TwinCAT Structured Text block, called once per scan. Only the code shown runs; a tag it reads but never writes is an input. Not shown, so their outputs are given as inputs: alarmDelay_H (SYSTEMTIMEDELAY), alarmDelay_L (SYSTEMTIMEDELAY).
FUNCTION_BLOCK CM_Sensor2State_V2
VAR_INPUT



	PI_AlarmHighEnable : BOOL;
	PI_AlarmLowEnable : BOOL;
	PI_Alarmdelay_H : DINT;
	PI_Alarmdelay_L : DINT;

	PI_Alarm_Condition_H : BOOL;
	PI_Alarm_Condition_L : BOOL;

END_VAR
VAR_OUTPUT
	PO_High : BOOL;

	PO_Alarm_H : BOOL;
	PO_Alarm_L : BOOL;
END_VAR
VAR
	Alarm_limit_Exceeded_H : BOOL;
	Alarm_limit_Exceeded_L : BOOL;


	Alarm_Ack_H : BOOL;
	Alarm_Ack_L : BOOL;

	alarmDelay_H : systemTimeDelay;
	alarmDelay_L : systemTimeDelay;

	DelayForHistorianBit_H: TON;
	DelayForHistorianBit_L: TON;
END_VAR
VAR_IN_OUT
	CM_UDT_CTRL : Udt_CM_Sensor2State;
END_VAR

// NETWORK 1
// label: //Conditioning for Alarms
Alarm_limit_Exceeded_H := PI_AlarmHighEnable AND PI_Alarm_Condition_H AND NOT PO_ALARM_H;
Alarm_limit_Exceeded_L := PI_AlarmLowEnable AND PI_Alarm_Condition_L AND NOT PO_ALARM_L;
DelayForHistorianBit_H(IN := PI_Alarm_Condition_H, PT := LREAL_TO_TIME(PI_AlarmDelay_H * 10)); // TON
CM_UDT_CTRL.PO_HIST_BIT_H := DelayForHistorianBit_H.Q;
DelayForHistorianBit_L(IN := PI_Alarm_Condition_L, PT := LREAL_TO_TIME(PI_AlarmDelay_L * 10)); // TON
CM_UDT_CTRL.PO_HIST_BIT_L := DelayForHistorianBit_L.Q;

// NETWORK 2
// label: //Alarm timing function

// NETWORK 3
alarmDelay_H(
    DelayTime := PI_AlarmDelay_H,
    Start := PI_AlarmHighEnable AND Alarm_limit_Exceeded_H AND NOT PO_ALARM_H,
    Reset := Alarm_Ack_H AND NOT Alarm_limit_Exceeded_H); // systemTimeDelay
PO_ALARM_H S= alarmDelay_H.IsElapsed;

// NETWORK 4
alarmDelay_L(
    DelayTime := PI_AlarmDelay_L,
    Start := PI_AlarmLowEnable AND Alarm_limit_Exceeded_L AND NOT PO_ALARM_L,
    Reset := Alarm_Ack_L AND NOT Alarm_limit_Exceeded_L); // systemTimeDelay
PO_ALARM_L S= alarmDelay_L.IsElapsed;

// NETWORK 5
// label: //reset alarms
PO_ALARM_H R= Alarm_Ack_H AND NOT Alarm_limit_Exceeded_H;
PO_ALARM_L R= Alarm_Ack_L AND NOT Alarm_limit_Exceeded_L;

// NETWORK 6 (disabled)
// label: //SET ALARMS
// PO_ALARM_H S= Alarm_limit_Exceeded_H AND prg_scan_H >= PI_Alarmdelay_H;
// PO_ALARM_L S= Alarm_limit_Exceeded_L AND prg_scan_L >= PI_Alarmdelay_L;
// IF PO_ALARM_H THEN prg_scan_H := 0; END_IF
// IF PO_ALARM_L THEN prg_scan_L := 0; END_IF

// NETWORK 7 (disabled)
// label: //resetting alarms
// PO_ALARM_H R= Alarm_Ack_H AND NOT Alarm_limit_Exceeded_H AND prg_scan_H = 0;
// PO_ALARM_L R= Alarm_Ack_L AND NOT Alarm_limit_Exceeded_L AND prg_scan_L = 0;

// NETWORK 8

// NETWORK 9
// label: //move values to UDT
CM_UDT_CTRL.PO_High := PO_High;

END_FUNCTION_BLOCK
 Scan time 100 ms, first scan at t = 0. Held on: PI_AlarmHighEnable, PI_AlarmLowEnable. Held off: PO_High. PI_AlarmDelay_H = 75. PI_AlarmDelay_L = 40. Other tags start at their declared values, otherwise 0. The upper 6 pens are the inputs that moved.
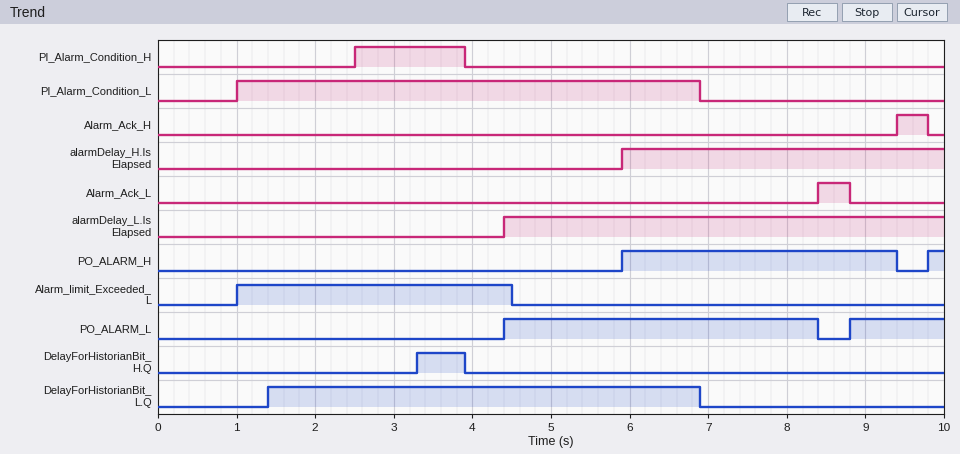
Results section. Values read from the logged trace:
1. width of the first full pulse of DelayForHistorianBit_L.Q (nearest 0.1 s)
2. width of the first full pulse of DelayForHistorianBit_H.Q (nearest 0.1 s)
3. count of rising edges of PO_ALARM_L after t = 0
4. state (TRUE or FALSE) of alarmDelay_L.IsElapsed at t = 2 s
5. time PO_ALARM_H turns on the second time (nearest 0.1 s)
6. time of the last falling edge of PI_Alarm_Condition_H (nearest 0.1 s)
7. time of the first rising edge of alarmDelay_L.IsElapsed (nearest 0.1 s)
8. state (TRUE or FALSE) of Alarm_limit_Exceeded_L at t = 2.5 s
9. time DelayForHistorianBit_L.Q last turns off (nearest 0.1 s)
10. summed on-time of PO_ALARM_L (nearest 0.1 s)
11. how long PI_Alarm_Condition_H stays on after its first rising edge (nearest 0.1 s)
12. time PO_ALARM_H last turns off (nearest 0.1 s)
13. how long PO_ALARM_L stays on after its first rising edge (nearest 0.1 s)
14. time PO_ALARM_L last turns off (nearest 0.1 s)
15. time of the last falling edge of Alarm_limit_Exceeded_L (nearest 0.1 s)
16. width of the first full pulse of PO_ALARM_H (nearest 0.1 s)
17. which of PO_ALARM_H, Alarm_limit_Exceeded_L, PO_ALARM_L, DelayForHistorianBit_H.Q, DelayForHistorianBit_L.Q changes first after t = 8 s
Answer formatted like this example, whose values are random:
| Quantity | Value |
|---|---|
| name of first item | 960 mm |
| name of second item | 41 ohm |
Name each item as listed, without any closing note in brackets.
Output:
| Quantity | Value |
|---|---|
| width of the first full pulse of DelayForHistorianBit_L.Q | 5.5 s |
| width of the first full pulse of DelayForHistorianBit_H.Q | 0.6 s |
| count of rising edges of PO_ALARM_L after t = 0 | 2 |
| state (TRUE or FALSE) of alarmDelay_L.IsElapsed at t = 2 s | FALSE |
| time PO_ALARM_H turns on the second time | 9.8 s |
| time of the last falling edge of PI_Alarm_Condition_H | 3.9 s |
| time of the first rising edge of alarmDelay_L.IsElapsed | 4.4 s |
| state (TRUE or FALSE) of Alarm_limit_Exceeded_L at t = 2.5 s | TRUE |
| time DelayForHistorianBit_L.Q last turns off | 6.9 s |
| summed on-time of PO_ALARM_L | 5.2 s |
| how long PI_Alarm_Condition_H stays on after its first rising edge | 1.4 s |
| time PO_ALARM_H last turns off | 9.4 s |
| how long PO_ALARM_L stays on after its first rising edge | 4.0 s |
| time PO_ALARM_L last turns off | 8.4 s |
| time of the last falling edge of Alarm_limit_Exceeded_L | 4.5 s |
| width of the first full pulse of PO_ALARM_H | 3.5 s |
| which of PO_ALARM_H, Alarm_limit_Exceeded_L, PO_ALARM_L, DelayForHistorianBit_H.Q, DelayForHistorianBit_L.Q changes first after t = 8 s | PO_ALARM_L |
